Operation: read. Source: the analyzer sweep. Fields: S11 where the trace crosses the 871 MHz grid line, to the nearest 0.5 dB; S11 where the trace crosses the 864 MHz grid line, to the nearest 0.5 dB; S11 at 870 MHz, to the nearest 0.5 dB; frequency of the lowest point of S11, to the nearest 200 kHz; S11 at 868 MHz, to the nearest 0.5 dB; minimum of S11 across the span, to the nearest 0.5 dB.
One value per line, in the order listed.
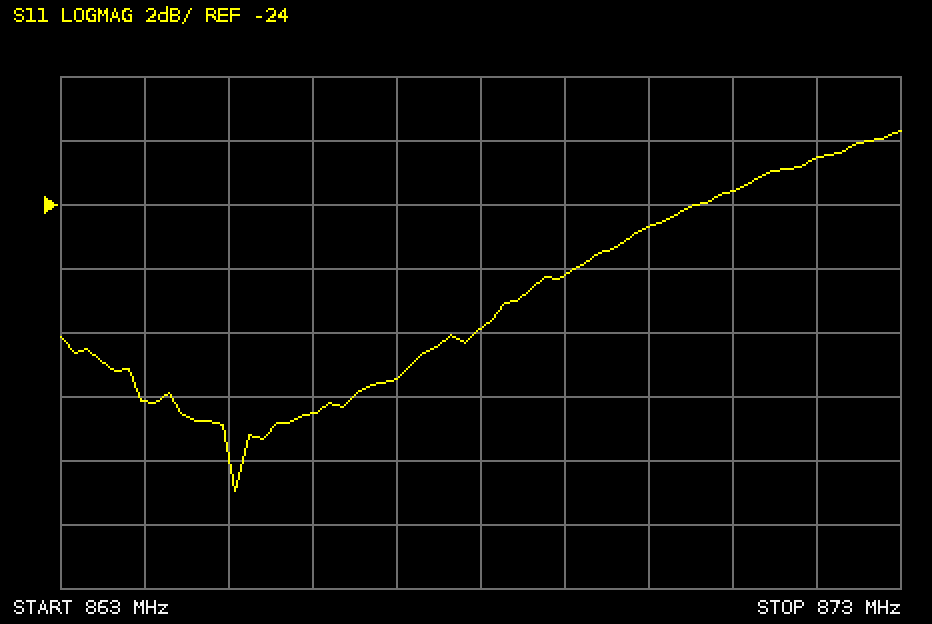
-23.5 dB
-30.0 dB
-24.5 dB
865.0 MHz
-28.0 dB
-33.0 dB
